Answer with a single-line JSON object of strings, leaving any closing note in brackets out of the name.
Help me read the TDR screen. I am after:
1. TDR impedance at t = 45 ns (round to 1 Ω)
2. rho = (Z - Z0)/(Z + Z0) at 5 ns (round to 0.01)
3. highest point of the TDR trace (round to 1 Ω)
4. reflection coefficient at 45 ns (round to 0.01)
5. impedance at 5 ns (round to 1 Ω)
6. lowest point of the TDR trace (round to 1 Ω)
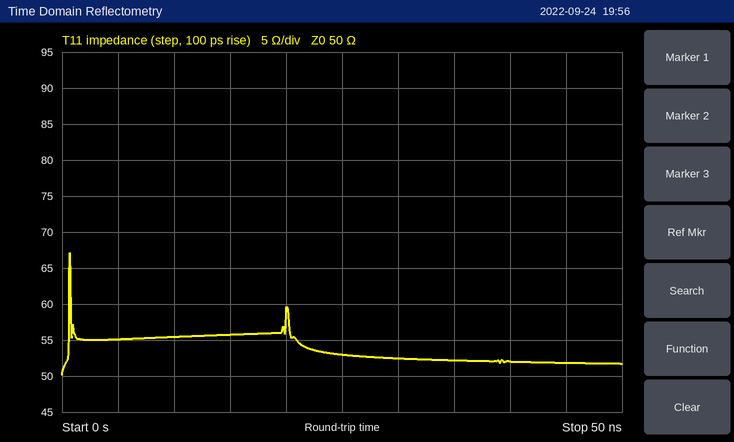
{"TDR impedance at t = 45 ns": "52 Ω", "rho = (Z - Z0)/(Z + Z0) at 5 ns": "+0.05", "highest point of the TDR trace": "67 Ω", "reflection coefficient at 45 ns": "+0.02", "impedance at 5 ns": "55 Ω", "lowest point of the TDR trace": "50 Ω"}
